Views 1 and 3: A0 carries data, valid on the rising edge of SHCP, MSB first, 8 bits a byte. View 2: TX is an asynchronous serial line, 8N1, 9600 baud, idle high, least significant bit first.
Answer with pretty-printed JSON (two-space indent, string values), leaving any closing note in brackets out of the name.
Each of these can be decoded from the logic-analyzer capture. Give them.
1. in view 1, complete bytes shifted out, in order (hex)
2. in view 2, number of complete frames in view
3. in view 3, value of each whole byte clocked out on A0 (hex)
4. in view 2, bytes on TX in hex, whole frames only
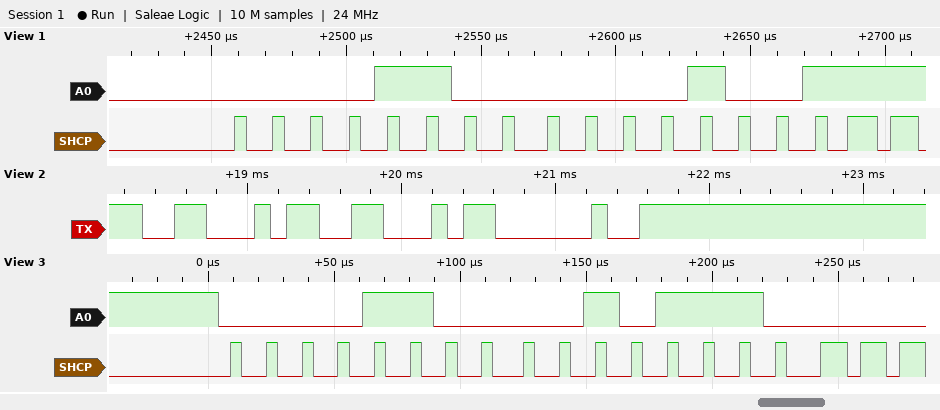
{
  "in view 1, complete bytes shifted out, in order": "0C 09",
  "in view 2, number of complete frames in view": "3",
  "in view 3, value of each whole byte clocked out on A0": "0x0C 0x2E",
  "in view 2, bytes on TX in hex, whole frames only": "0x46 0x46 0x20"
}
